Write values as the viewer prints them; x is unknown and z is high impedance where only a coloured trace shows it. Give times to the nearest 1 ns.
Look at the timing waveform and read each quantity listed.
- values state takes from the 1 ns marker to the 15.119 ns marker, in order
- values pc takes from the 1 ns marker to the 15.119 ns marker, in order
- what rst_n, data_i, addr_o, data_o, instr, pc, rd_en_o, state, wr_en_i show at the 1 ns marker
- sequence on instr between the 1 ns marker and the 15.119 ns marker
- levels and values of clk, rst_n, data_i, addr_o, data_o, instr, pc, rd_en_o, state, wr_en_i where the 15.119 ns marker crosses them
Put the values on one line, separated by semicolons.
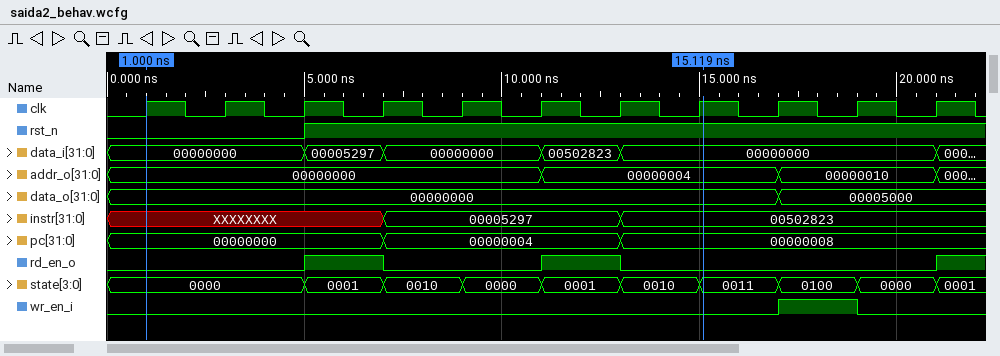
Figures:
0000, 0001, 0010, 0000, 0001, 0010, 0011; 00000000, 00000004, 00000008; rst_n=0, data_i=00000000, addr_o=00000000, data_o=00000000, instr=XXXXXXXX, pc=00000000, rd_en_o=0, state=0000, wr_en_i=0; XXXXXXXX, 00005297, 00502823; clk=1, rst_n=1, data_i=00000000, addr_o=00000004, data_o=00000000, instr=00502823, pc=00000008, rd_en_o=0, state=0011, wr_en_i=0
